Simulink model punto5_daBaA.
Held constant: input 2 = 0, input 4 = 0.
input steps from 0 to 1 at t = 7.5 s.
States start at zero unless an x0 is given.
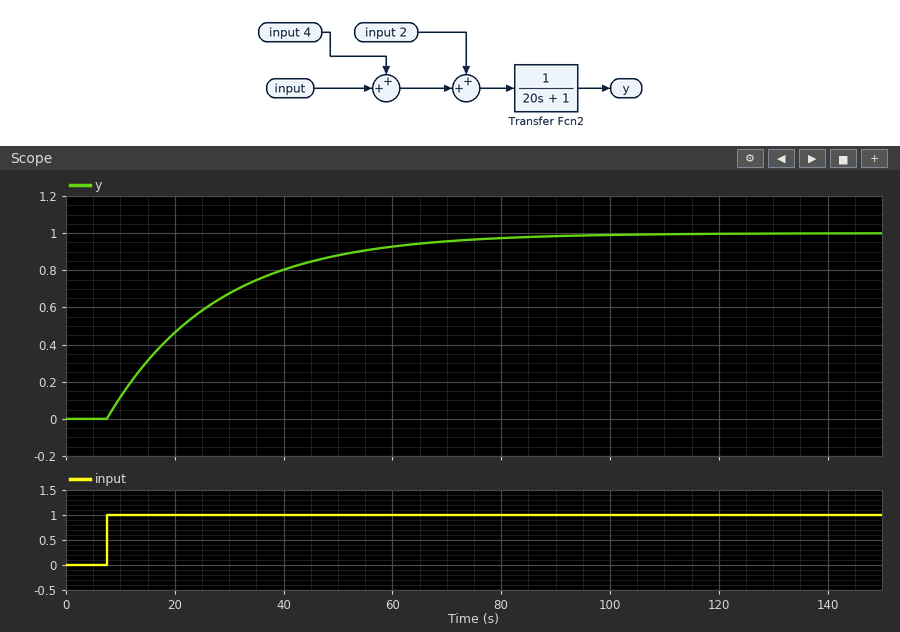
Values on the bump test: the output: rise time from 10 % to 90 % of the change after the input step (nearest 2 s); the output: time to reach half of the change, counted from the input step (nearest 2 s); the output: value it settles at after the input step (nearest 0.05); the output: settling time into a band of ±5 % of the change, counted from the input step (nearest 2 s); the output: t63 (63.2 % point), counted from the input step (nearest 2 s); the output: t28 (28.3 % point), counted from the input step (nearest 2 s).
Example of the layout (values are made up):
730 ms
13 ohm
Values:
44 s
14 s
1.00
60 s
20 s
6 s
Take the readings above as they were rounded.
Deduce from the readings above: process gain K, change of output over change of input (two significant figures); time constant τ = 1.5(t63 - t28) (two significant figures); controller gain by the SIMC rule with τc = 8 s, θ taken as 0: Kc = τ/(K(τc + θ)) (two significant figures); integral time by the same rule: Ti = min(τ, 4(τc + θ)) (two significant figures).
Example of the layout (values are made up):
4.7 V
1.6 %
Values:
1.0
21 s
2.6
21 s
